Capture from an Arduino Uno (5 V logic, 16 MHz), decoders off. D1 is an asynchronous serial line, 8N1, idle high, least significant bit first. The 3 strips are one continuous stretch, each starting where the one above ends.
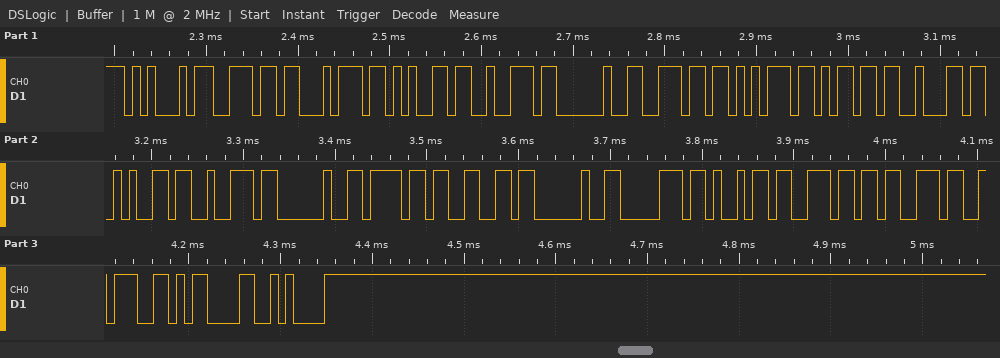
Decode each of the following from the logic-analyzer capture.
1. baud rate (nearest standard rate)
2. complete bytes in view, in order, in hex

115200 baud
45 6E 74 65 72 20 6E 75 6D 62 65 72 20 6F 66 20 70 69 6E 73 3A 0D 0A
